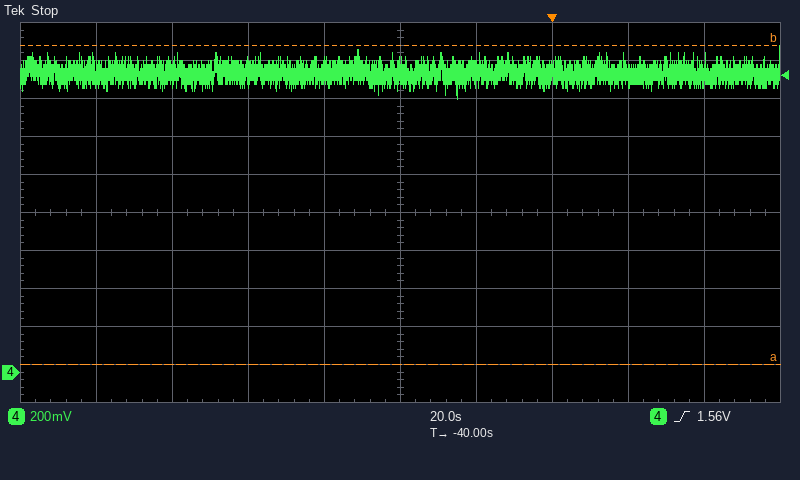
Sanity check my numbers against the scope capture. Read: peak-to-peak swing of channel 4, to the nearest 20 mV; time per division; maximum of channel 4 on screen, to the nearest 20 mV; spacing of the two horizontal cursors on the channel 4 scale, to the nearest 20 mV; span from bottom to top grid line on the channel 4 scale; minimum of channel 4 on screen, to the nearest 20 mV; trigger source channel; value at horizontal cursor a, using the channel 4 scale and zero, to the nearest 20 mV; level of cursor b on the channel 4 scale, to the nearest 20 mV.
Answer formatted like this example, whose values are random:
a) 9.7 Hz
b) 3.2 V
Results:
a) 280 mV
b) 20 s
c) 1.72 V
d) 1.68 V
e) 2 V
f) 1.44 V
g) channel 4
h) 40 mV
i) 1.72 V
